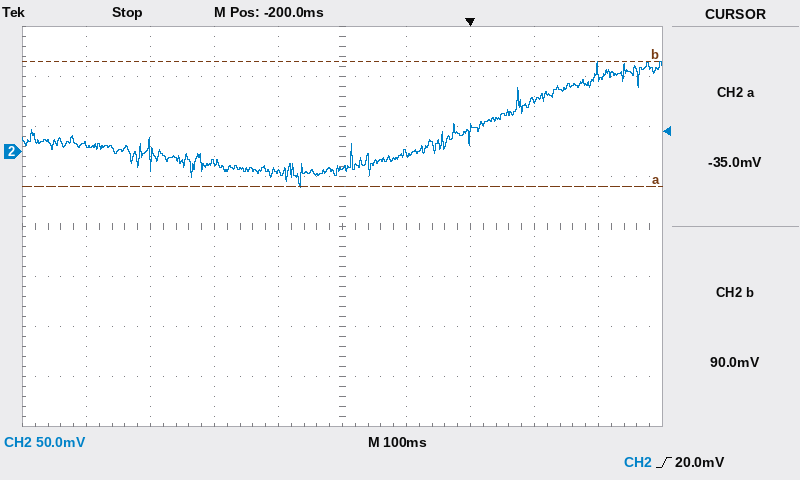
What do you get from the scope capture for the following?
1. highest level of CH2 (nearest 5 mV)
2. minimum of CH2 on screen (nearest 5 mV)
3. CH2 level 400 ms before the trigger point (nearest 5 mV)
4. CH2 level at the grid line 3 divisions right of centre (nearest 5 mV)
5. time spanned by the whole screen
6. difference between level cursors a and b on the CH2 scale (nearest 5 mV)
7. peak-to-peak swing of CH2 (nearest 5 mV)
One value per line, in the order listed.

90 mV
-35 mV
-10 mV
50 mV
1 s
125 mV
125 mV
